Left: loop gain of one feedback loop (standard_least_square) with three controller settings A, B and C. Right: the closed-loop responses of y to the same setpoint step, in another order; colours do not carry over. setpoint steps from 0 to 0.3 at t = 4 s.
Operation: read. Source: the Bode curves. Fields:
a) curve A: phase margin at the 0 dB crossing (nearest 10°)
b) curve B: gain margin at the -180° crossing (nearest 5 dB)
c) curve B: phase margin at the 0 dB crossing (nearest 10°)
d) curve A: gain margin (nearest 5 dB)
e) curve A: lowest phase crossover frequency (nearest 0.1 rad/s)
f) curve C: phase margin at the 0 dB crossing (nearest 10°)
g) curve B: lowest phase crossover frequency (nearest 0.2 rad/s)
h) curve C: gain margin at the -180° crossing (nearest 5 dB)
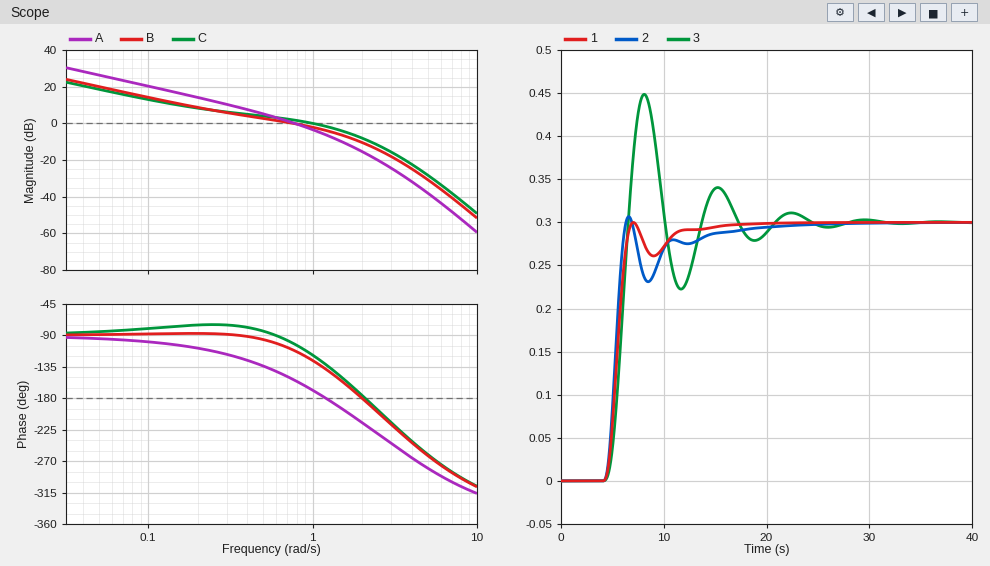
30°
10 dB
70°
5 dB
1.2 rad/s
60°
2.0 rad/s
10 dB
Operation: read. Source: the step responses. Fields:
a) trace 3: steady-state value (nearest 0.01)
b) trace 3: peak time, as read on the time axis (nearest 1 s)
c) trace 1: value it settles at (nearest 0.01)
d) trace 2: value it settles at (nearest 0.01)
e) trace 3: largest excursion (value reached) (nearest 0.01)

0.30
8 s
0.30
0.30
0.45
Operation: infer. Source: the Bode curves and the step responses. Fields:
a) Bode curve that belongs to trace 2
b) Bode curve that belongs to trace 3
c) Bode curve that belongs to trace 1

C
A
B
